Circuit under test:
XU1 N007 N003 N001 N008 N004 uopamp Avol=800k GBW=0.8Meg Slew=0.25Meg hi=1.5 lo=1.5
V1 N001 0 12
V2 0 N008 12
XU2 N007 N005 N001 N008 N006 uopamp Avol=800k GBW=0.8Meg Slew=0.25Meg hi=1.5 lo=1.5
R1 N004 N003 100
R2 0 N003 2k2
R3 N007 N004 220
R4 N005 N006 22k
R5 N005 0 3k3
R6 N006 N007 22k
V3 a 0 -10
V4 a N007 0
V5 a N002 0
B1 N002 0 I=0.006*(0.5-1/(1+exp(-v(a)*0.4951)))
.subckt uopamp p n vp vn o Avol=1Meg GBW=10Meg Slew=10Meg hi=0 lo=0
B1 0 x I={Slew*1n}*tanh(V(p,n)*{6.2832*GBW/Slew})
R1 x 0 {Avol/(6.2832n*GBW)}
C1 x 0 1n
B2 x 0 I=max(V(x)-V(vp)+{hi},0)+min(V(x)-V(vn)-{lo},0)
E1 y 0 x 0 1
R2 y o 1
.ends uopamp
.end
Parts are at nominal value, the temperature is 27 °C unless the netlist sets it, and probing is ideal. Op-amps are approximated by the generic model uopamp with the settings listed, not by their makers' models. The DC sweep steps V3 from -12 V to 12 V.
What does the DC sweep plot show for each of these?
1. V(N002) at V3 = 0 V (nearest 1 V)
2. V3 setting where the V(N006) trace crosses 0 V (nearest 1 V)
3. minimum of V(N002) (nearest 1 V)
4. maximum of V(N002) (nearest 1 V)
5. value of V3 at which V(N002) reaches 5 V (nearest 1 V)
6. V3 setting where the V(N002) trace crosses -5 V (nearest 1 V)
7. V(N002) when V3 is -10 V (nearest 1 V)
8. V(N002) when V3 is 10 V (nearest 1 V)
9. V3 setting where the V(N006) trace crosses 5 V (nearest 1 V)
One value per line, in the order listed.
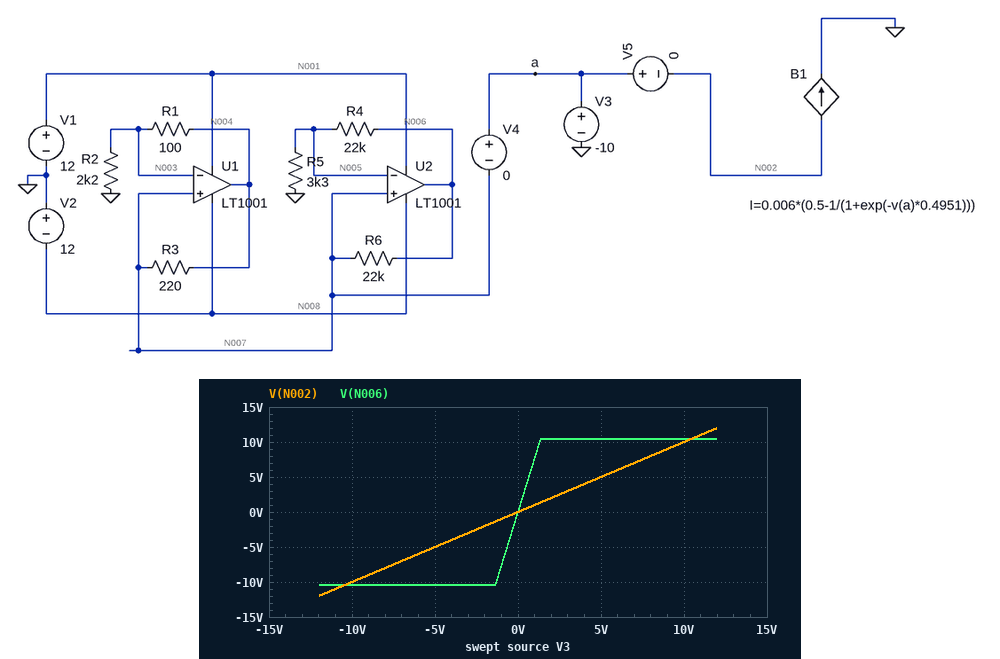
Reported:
0 V
0 V
-12 V
12 V
5 V
-5 V
-10 V
10 V
1 V
